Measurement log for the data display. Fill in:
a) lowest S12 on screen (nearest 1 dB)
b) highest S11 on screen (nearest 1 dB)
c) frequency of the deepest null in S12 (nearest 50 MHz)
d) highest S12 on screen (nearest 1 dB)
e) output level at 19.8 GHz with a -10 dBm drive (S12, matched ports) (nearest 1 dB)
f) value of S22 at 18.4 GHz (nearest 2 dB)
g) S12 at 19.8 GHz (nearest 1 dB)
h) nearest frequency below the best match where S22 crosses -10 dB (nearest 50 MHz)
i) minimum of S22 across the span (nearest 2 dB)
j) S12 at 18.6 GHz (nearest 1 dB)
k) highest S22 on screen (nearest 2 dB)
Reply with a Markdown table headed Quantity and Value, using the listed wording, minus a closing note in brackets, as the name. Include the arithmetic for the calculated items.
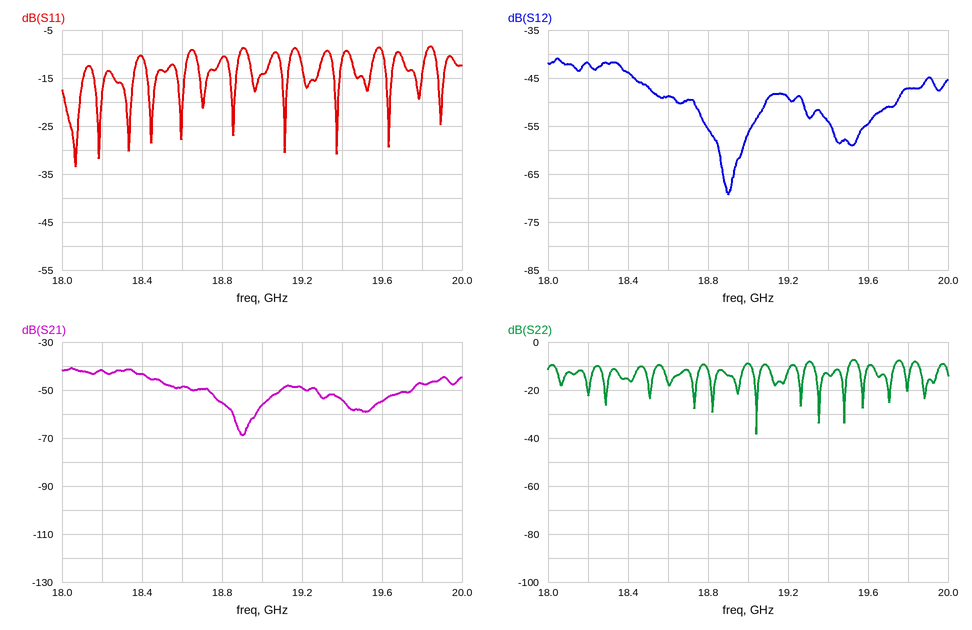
| Quantity | Value |
|---|---|
| lowest S12 on screen | -69 dB |
| highest S11 on screen | -8 dB |
| frequency of the deepest null in S12 | 18.90 GHz |
| highest S12 on screen | -41 dB |
| output level at 19.8 GHz with a -10 dBm drive (S12, matched ports) | -10 dBm + (-47 dB) = -57 dBm |
| value of S22 at 18.4 GHz | -16 dB |
| S12 at 19.8 GHz | -47 dB |
| nearest frequency below the best match where S22 crosses -10 dB | 19.00 GHz |
| minimum of S22 across the span | -38 dB |
| S12 at 18.6 GHz | -49 dB |
| highest S22 on screen | -8 dB |
